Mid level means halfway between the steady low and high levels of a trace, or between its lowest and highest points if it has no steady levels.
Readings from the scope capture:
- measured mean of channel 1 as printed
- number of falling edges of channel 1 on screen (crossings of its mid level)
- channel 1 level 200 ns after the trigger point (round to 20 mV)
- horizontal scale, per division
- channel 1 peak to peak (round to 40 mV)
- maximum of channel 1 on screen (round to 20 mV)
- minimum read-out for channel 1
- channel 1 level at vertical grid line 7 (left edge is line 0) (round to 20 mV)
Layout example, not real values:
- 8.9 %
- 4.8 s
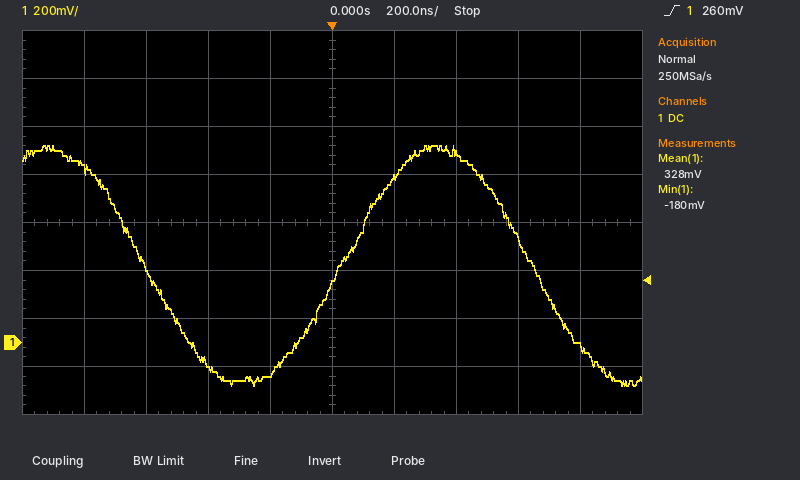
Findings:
- 328 mV
- 2
- 680 mV
- 200 ns
- 1.00 V
- 820 mV
- -180 mV
- 800 mV
